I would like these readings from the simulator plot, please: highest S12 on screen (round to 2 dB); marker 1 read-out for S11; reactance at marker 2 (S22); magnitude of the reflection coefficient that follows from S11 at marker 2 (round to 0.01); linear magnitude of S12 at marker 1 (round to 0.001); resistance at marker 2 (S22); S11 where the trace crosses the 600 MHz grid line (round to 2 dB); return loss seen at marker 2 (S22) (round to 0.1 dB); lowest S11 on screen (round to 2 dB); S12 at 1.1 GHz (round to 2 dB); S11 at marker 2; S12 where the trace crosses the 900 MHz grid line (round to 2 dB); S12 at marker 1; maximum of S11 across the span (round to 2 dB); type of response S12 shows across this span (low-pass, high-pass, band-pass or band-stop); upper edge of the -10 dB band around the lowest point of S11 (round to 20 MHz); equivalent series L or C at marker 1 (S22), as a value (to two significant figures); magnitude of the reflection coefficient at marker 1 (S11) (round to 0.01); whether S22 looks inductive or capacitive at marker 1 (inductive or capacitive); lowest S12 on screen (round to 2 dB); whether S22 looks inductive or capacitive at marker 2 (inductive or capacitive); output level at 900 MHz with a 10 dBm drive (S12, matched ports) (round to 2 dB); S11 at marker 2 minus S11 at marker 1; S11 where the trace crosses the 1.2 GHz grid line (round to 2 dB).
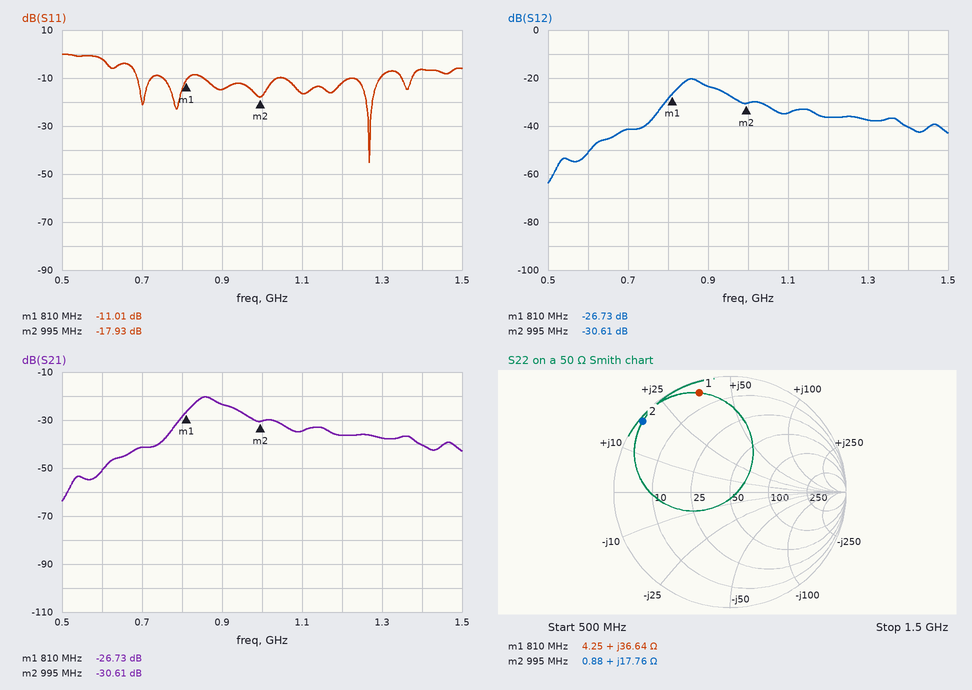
-20 dB
-11.01 dB
+17.76 Ω
0.13
0.046
0.88 Ω
-2 dB
0.3 dB
-46 dB
-34 dB
-17.93 dB
-24 dB
-26.73 dB
0 dB
band-pass
1.30 GHz
7.2 nH
0.28
inductive
-64 dB
inductive
-14 dBm
-6.92 dB
-12 dB
